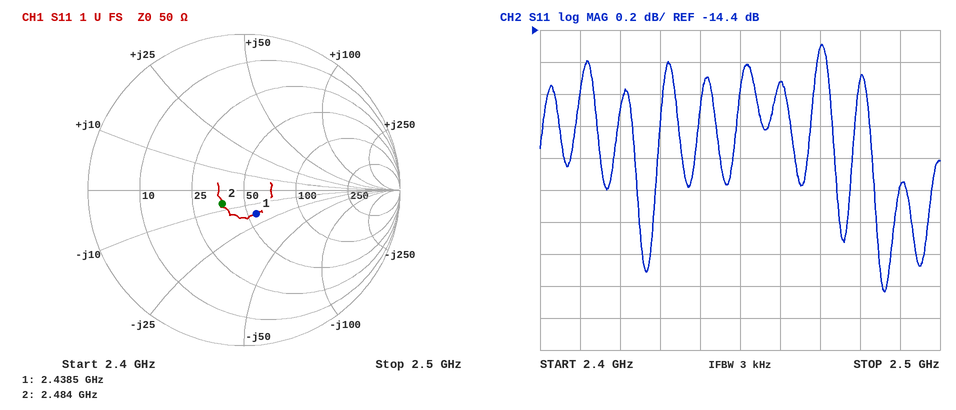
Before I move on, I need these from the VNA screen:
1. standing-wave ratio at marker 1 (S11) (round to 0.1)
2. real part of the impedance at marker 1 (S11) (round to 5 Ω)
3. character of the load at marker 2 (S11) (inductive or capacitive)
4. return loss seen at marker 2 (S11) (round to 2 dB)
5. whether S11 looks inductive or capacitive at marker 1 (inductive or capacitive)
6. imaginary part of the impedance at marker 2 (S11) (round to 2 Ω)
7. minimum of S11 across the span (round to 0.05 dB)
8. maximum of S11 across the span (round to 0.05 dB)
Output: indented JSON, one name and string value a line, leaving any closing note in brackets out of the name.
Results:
{
  "standing-wave ratio at marker 1 (S11)": "1.4",
  "real part of the impedance at marker 1 (S11)": "55 Ω",
  "character of the load at marker 2 (S11)": "capacitive",
  "return loss seen at marker 2 (S11)": "16 dB",
  "whether S11 looks inductive or capacitive at marker 1": "capacitive",
  "imaginary part of the impedance at marker 2 (S11)": "-6 Ω",
  "minimum of S11 across the span": "-16.05 dB",
  "maximum of S11 across the span": "-14.50 dB"
}
